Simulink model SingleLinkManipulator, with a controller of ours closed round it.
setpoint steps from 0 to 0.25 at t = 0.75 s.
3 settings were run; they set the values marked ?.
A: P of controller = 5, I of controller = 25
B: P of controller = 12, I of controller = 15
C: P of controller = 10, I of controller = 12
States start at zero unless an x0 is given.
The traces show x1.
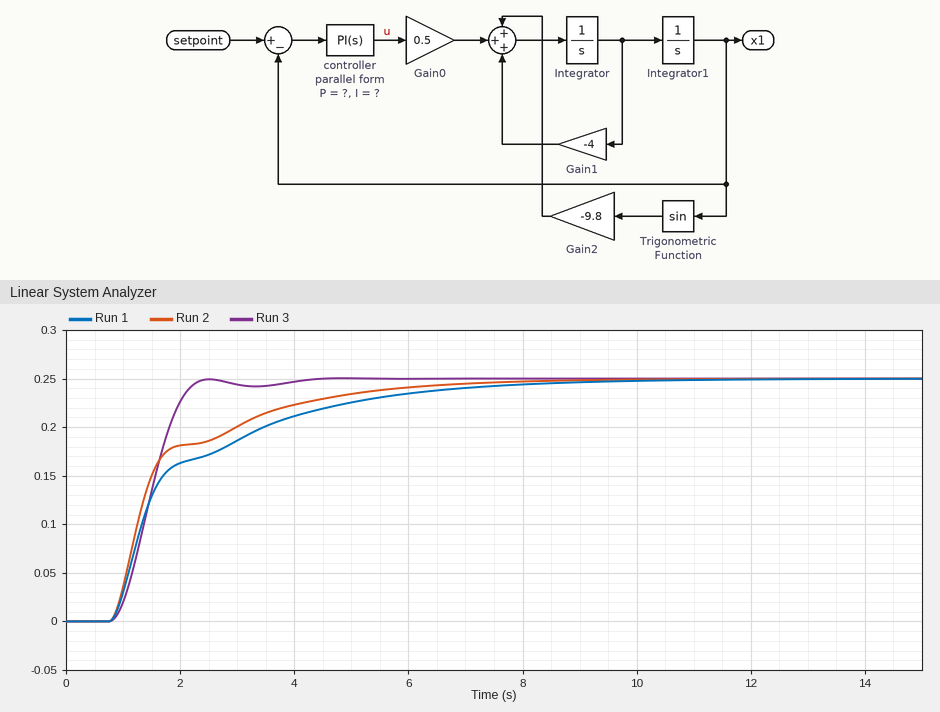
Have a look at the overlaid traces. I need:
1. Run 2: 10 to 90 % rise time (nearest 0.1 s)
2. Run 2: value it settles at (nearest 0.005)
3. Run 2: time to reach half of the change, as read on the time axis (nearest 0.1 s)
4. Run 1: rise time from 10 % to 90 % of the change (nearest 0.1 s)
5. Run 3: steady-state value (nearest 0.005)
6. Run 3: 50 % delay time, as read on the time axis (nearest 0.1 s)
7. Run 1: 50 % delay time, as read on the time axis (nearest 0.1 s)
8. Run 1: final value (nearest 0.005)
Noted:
3.2 s
0.250
1.4 s
4.0 s
0.250
1.5 s
1.5 s
0.250
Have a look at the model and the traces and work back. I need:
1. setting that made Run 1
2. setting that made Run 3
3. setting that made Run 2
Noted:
C
A
B
